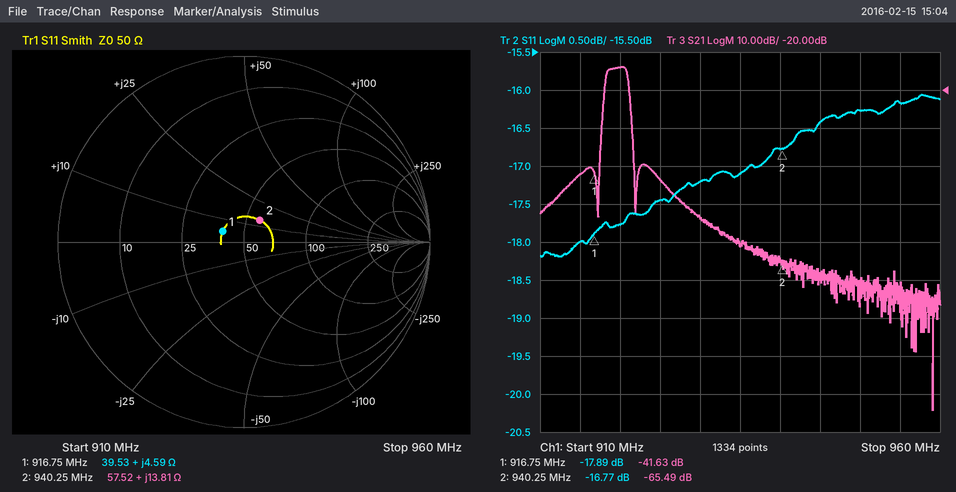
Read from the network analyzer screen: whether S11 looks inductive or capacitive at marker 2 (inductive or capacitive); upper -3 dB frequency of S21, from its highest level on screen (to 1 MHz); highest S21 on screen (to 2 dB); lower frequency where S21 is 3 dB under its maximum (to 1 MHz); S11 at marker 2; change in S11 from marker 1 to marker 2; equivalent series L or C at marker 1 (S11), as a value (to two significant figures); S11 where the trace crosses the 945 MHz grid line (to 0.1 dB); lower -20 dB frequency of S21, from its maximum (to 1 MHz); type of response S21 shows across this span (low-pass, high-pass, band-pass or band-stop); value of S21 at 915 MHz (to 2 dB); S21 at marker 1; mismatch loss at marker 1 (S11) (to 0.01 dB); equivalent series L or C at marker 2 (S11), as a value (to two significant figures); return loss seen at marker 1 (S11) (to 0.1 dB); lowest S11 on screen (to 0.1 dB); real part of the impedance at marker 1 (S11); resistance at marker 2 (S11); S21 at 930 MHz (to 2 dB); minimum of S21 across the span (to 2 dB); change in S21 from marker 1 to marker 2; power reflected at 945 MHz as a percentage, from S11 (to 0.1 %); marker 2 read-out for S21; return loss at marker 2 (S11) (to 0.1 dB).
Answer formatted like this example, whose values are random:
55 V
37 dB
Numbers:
inductive
921 MHz
-14 dB
918 MHz
-16.77 dB
1.12 dB
800 pH
-16.4 dB
918 MHz
band-pass
-42 dB
-41.63 dB
0.07 dB
2.3 nH
17.9 dB
-18.2 dB
39.53 Ω
57.52 Ω
-54 dB
-104 dB
-23.86 dB
2.3 %
-65.49 dB
16.8 dB
